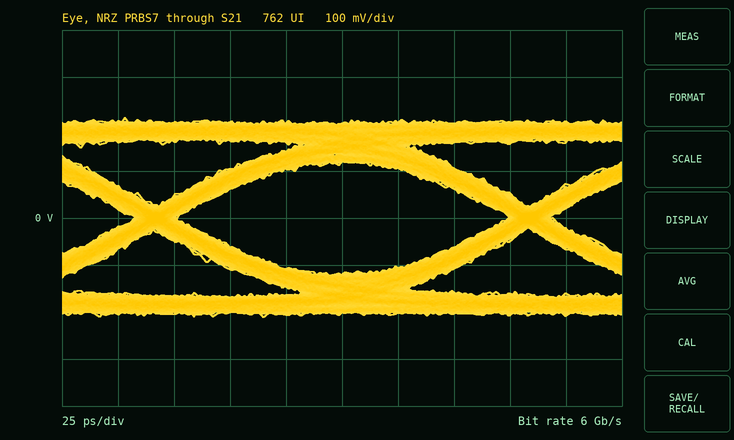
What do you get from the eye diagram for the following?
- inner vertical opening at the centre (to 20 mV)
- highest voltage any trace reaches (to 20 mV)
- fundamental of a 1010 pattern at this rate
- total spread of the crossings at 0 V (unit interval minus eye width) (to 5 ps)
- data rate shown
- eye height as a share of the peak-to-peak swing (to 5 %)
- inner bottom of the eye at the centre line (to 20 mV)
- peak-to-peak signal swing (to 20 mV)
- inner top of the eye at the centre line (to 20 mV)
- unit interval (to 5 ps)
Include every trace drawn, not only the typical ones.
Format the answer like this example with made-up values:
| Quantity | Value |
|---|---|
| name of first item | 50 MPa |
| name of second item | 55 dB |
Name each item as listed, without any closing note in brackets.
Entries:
| Quantity | Value |
|---|---|
| inner vertical opening at the centre | 240 mV |
| highest voltage any trace reaches | 220 mV |
| fundamental of a 1010 pattern at this rate | 3 GHz |
| total spread of the crossings at 0 V (unit interval minus eye width) | 20 ps |
| data rate shown | 6 Gb/s |
| eye height as a share of the peak-to-peak swing | 55 % |
| inner bottom of the eye at the centre line | -120 mV |
| peak-to-peak signal swing | 420 mV |
| inner top of the eye at the centre line | 120 mV |
| unit interval | 165 ps |
